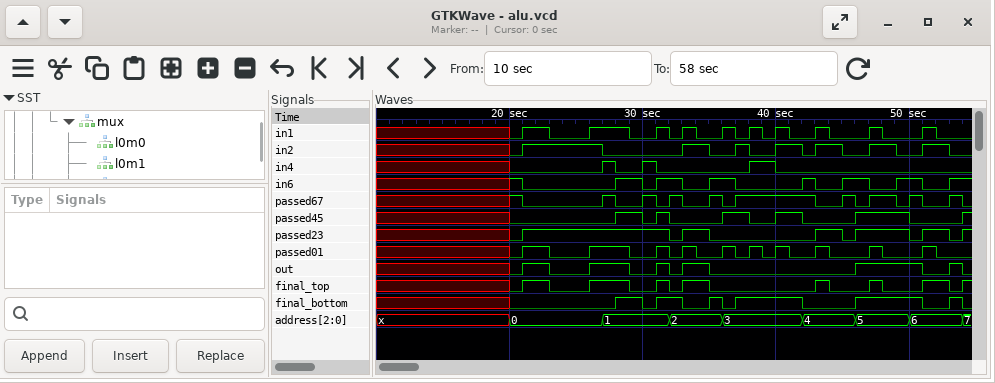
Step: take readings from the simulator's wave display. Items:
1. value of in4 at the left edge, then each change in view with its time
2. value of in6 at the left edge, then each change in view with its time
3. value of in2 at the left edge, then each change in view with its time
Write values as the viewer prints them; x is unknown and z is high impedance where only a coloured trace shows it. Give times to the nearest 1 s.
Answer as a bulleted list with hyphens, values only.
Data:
- x, 0 at 20 s, 1 at 27 s, 0 at 28 s, 1 at 30 s, 0 at 31 s, 1 at 38 s, 0 at 40 s
- x, 1 at 20 s, 0 at 21 s, 1 at 28 s, 0 at 30 s, 1 at 31 s, 0 at 33 s, 1 at 35 s, 0 at 37 s, 1 at 42 s, 0 at 43 s, 1 at 45 s, 0 at 47 s, 1 at 49 s, 0 at 51 s, 1 at 53 s
- x, 0 at 20 s, 1 at 21 s, 0 at 27 s, 1 at 33 s, 0 at 35 s, 1 at 37 s, 0 at 38 s, 1 at 40 s, 0 at 42 s, 1 at 43 s, 0 at 45 s, 1 at 47 s, 0 at 49 s, 1 at 51 s, 0 at 53 s
